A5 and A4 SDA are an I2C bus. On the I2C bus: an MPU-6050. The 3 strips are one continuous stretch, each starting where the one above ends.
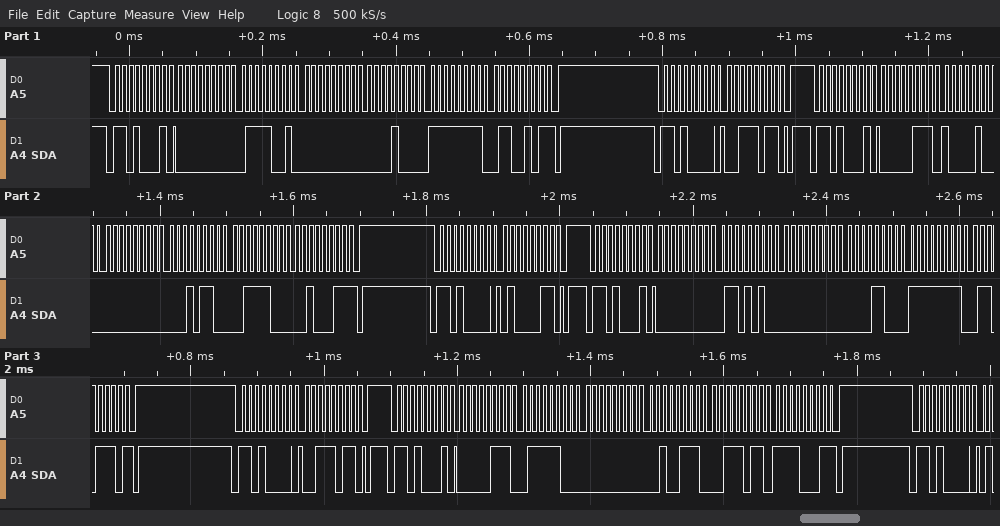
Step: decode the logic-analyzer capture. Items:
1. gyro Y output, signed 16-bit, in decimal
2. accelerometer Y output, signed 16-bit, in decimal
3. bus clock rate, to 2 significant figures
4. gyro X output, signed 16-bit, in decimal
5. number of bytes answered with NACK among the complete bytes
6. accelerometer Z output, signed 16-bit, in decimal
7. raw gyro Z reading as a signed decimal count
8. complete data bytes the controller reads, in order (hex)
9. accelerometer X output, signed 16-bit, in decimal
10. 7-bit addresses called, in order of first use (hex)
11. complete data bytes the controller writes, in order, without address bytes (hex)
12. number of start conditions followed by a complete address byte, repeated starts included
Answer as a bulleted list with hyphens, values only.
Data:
- 12
- 22
- 100 kHz
- 106
- 4
- 15395
- -146
- 00 79 00 08 FF 65 07 84 00 16 3C 23 00 6A 00 0C FF 6E 07 7C 00 27 3B F1
- 1924
- 0x68
- 3B 43 3B
- 8
